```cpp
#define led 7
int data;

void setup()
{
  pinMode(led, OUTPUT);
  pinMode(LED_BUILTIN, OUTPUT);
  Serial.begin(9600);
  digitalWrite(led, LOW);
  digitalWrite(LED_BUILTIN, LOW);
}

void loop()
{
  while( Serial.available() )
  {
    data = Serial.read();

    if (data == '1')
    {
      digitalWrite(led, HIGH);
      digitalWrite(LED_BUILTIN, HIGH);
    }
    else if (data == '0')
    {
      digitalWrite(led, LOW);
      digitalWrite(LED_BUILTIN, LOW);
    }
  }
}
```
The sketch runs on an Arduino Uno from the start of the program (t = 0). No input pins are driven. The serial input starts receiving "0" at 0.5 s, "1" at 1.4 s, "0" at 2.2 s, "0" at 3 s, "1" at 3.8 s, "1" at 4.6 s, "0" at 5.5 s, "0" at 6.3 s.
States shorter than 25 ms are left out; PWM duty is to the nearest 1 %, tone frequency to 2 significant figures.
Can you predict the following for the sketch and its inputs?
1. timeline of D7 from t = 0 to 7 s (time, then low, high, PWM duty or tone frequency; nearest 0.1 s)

0 s low; 1.4 s high; 2.2 s low; 3.8 s high; 5.5 s low
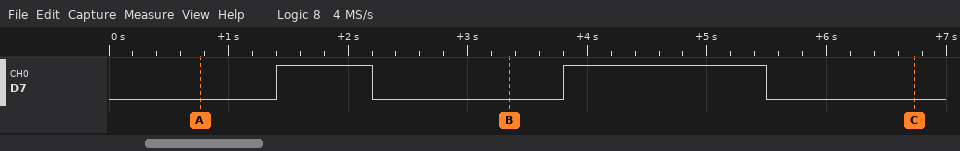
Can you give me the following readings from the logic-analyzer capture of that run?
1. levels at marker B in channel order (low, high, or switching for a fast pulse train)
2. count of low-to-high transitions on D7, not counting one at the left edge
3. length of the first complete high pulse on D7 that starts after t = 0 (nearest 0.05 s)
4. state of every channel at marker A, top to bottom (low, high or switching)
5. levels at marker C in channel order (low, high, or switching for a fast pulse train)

D7 low
2
0.80 s
D7 low
D7 low
